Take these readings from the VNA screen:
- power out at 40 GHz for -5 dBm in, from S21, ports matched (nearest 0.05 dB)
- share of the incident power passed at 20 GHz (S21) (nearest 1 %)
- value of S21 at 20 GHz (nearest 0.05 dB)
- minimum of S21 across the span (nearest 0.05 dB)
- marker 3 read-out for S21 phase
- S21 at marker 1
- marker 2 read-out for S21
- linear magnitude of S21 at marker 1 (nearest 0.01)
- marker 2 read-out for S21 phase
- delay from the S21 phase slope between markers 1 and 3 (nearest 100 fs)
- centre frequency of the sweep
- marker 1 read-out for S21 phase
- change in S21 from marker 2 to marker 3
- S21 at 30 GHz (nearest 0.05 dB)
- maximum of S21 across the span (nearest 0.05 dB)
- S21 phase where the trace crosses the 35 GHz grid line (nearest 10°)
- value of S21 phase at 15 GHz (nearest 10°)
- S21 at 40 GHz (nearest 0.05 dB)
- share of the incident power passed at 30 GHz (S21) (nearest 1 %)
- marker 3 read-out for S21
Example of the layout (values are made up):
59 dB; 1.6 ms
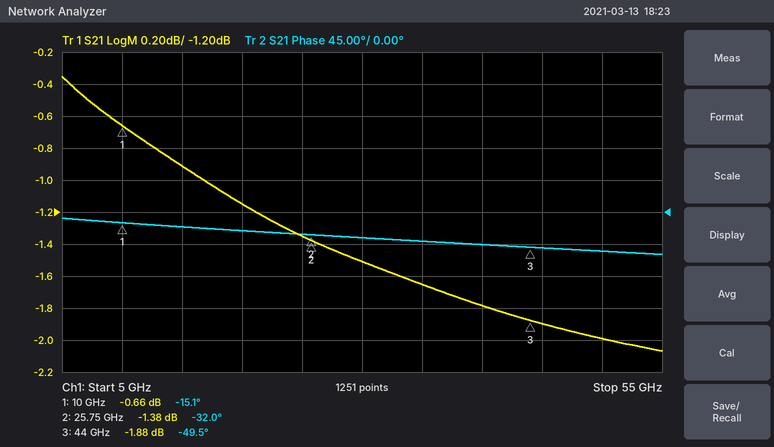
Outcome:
-6.80 dBm; 77 %; -1.15 dB; -2.05 dB; -49.5°; -0.66 dB; -1.38 dB; 0.93; -32.0°; 2.8 ps; 30 GHz; -15.1°; -0.50 dB; -1.50 dB; -0.35 dB; -40°; -20°; -1.80 dB; 71 %; -1.88 dB
